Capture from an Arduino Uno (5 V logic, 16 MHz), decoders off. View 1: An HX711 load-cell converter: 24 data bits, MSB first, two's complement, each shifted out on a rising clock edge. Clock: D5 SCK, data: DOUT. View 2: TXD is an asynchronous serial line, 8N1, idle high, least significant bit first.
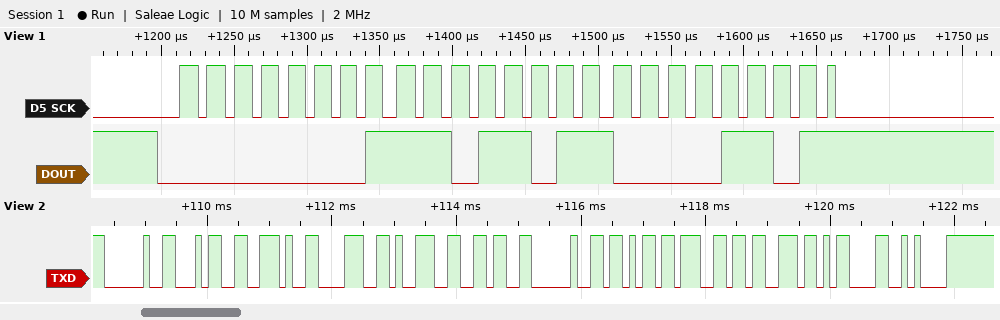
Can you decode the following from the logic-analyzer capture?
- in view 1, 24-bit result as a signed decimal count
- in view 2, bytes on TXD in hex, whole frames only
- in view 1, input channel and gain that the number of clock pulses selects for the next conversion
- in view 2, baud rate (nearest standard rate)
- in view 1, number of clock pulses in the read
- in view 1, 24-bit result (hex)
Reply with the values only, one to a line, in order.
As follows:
121613
0x20 0x34 0x2E 0x38 0x39 0x36 0x20 0x6B 0x67 0x73 0x0D 0x0A
channel A, gain 128
9600 baud
25
0x01DB0D
